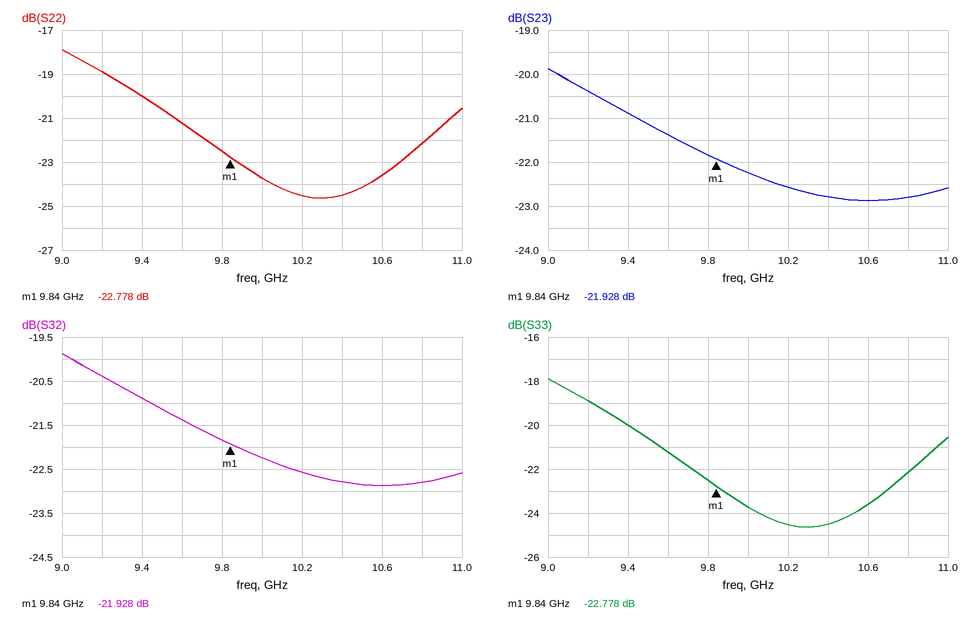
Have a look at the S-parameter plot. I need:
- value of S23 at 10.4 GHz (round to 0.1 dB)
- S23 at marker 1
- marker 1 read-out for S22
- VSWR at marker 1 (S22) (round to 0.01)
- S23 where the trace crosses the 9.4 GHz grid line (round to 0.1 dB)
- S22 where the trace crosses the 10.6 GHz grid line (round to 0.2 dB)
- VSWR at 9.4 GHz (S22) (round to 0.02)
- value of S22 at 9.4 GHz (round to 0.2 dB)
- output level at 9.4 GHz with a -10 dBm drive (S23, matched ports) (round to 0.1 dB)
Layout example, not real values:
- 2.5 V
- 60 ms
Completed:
- -22.8 dB
- -21.928 dB
- -22.778 dB
- 1.16
- -20.9 dB
- -23.6 dB
- 1.22
- -20.0 dB
- -30.9 dBm
